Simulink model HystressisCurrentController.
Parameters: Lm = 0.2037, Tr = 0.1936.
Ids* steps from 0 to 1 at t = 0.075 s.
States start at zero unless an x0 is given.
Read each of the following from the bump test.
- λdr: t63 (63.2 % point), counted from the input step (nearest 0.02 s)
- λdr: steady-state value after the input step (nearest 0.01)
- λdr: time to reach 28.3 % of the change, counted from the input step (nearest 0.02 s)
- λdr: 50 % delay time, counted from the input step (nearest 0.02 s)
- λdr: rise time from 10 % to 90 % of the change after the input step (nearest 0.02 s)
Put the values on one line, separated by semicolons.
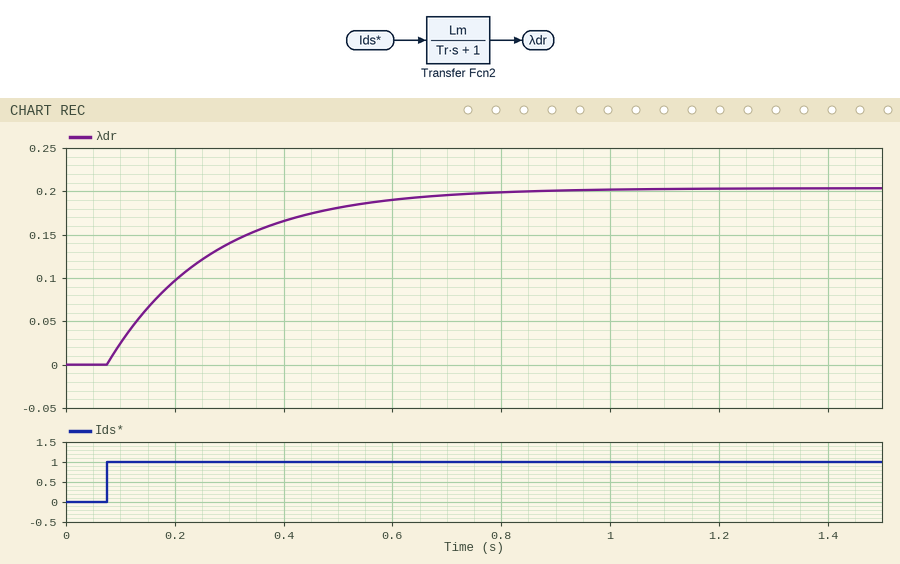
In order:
0.20 s; 0.20; 0.06 s; 0.14 s; 0.42 s
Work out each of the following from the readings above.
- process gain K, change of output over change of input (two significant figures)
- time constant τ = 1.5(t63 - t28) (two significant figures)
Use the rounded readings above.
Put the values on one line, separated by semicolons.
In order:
0.20; 0.21 s
